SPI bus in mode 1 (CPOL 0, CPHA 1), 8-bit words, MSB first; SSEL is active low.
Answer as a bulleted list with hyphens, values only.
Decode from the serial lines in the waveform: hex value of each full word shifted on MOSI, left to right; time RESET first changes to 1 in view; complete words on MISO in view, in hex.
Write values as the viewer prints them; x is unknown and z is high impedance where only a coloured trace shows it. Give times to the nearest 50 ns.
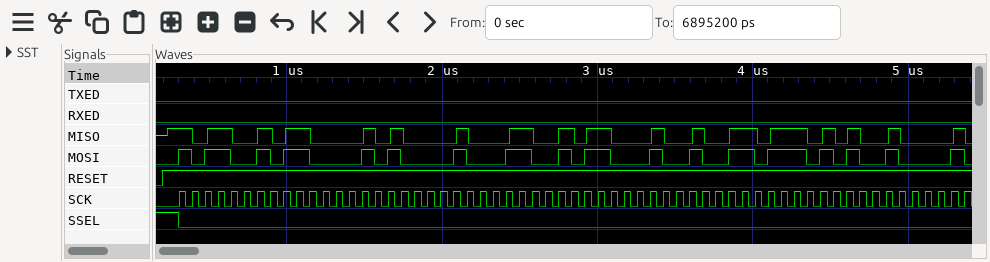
- B2, C2, 84, 65, 89, 37, 52
- 200 ns
- B2, C2, 84, 65, 89, 37, 52
